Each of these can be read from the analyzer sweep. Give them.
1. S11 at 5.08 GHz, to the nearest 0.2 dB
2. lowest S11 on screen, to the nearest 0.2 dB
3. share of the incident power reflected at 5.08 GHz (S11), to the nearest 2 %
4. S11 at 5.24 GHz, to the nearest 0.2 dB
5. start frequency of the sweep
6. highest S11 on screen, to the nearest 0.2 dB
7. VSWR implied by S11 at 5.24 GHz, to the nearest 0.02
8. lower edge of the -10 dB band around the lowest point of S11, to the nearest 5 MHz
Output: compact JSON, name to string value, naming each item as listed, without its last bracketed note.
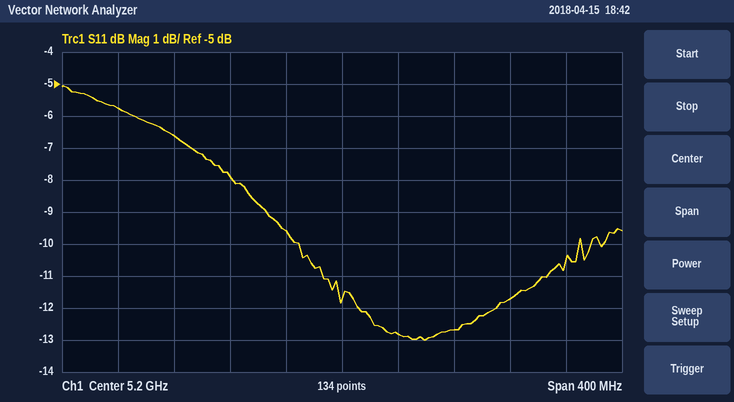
{"S11 at 5.08 GHz, to the nearest 0.2 dB": "-6.6 dB", "lowest S11 on screen, to the nearest 0.2 dB": "-13.0 dB", "share of the incident power reflected at 5.08 GHz (S11), to the nearest 2 %": "22 %", "S11 at 5.24 GHz, to the nearest 0.2 dB": "-12.8 dB", "start frequency of the sweep": "5 GHz", "highest S11 on screen, to the nearest 0.2 dB": "-5.0 dB", "VSWR implied by S11 at 5.24 GHz, to the nearest 0.02": "1.60", "lower edge of the -10 dB band around the lowest point of S11, to the nearest 5 MHz": "5.170 GHz"}
